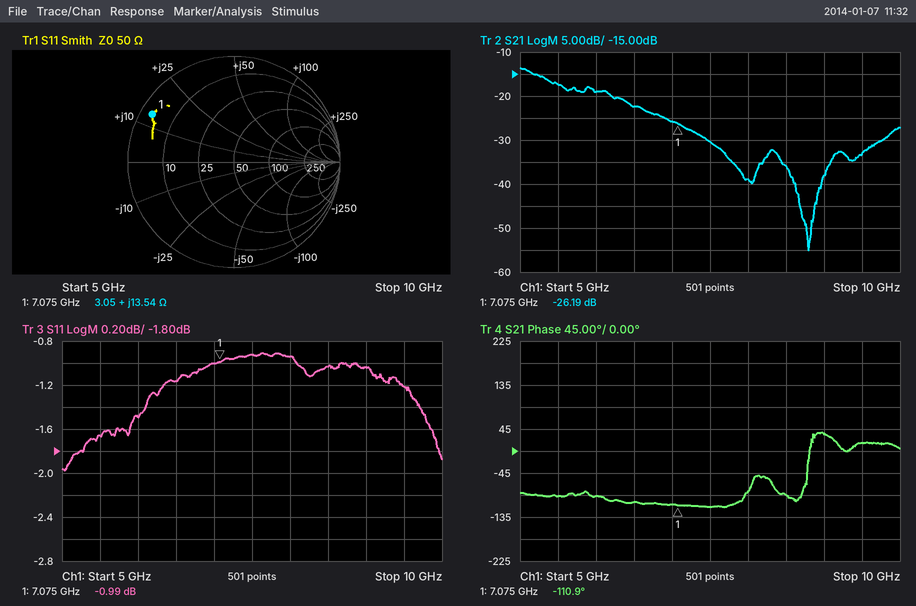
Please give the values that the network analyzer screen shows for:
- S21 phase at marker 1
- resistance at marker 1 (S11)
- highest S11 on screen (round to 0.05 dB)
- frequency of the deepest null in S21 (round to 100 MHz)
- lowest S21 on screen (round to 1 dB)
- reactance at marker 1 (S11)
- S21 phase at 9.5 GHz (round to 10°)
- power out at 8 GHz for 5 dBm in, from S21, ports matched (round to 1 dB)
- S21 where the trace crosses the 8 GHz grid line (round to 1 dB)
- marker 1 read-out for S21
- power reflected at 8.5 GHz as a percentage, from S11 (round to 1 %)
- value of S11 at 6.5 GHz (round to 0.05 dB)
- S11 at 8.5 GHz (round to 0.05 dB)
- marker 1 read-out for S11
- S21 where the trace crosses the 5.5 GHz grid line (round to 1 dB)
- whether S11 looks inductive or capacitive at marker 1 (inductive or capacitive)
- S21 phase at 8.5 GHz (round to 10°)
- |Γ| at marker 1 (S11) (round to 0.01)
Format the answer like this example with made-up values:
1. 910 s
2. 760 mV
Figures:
1. -110.9°
2. 3.05 Ω
3. -0.90 dB
4. 8.8 GHz
5. -55 dB
6. +13.54 Ω
7. 20°
8. -34 dBm
9. -39 dB
10. -26.19 dB
11. 79 %
12. -1.15 dB
13. -1.05 dB
14. -0.99 dB
15. -17 dB
16. inductive
17. -90°
18. 0.89
